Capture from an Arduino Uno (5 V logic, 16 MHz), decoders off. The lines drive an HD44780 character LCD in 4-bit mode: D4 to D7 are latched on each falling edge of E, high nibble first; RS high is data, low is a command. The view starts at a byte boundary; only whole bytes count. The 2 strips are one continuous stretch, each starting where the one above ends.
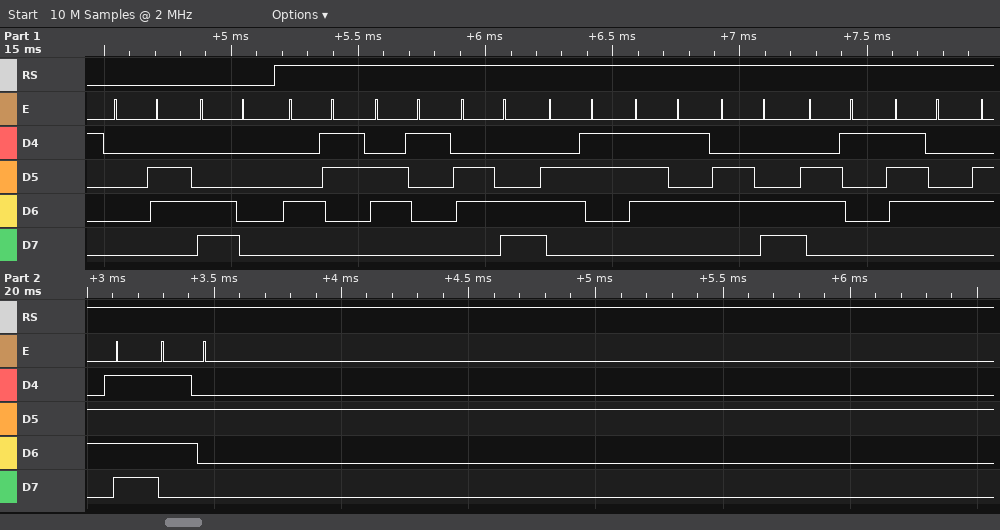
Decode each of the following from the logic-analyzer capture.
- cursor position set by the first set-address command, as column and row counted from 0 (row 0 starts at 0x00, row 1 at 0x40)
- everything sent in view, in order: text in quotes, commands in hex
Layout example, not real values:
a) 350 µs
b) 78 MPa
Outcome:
a) column 0, row 1
b) 0x06 0xC0 "Calculator"
